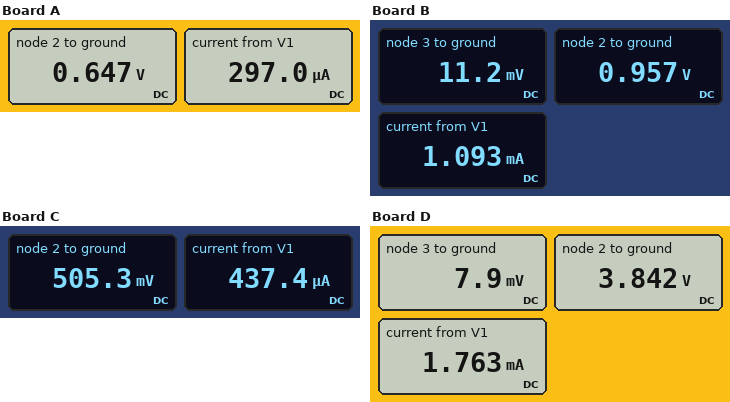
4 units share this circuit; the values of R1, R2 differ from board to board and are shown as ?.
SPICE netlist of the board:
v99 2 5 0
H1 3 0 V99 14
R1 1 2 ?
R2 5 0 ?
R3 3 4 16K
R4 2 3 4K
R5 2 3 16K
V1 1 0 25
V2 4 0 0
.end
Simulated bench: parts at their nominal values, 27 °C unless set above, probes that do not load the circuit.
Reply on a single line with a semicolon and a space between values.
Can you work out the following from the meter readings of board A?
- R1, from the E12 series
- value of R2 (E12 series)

82 kΩ; 6.8 kΩ
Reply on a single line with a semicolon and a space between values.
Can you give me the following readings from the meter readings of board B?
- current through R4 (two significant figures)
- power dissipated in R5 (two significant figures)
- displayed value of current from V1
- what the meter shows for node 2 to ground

240 µA; 56 µW; 1.093 mA; 0.957 V
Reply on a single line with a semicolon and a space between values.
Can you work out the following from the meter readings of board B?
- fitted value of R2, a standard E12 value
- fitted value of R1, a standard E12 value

1.2 kΩ; 22 kΩ
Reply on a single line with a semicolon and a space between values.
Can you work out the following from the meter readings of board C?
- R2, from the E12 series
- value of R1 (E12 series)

1.8 kΩ; 56 kΩ
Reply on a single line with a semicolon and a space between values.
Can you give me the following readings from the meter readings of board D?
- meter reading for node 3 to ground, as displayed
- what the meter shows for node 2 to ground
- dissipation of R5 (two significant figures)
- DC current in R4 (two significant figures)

7.9 mV; 3.842 V; 920 µW; 960 µA
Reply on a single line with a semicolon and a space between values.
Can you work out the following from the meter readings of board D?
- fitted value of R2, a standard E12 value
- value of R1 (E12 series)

6.8 kΩ; 12 kΩ
